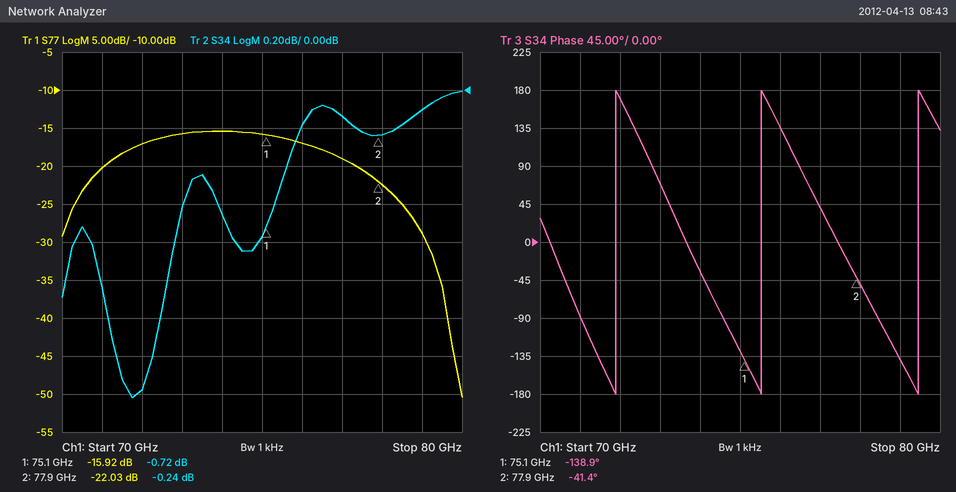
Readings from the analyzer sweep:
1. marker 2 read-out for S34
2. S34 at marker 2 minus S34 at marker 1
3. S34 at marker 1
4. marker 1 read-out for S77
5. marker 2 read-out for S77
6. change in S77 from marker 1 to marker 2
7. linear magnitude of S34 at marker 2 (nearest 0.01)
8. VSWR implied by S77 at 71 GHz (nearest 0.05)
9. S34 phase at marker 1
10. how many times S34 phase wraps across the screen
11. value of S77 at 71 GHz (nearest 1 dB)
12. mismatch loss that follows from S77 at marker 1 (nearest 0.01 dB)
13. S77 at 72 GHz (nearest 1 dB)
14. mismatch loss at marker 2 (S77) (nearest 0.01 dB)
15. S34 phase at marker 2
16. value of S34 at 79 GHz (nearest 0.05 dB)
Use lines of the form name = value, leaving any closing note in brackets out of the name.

marker 2 read-out for S34 = -0.24 dB
S34 at marker 2 minus S34 at marker 1 = 0.48 dB
S34 at marker 1 = -0.72 dB
marker 1 read-out for S77 = -15.92 dB
marker 2 read-out for S77 = -22.03 dB
change in S77 from marker 1 to marker 2 = -6.11 dB
linear magnitude of S34 at marker 2 = 0.97
VSWR implied by S77 at 71 GHz = 1.20
S34 phase at marker 1 = -138.9°
how many times S34 phase wraps across the screen = 3
value of S77 at 71 GHz = -20 dB
mismatch loss that follows from S77 at marker 1 = 0.11 dB
S77 at 72 GHz = -17 dB
mismatch loss at marker 2 (S77) = 0.03 dB
S34 phase at marker 2 = -41.4°
value of S34 at 79 GHz = -0.10 dB
